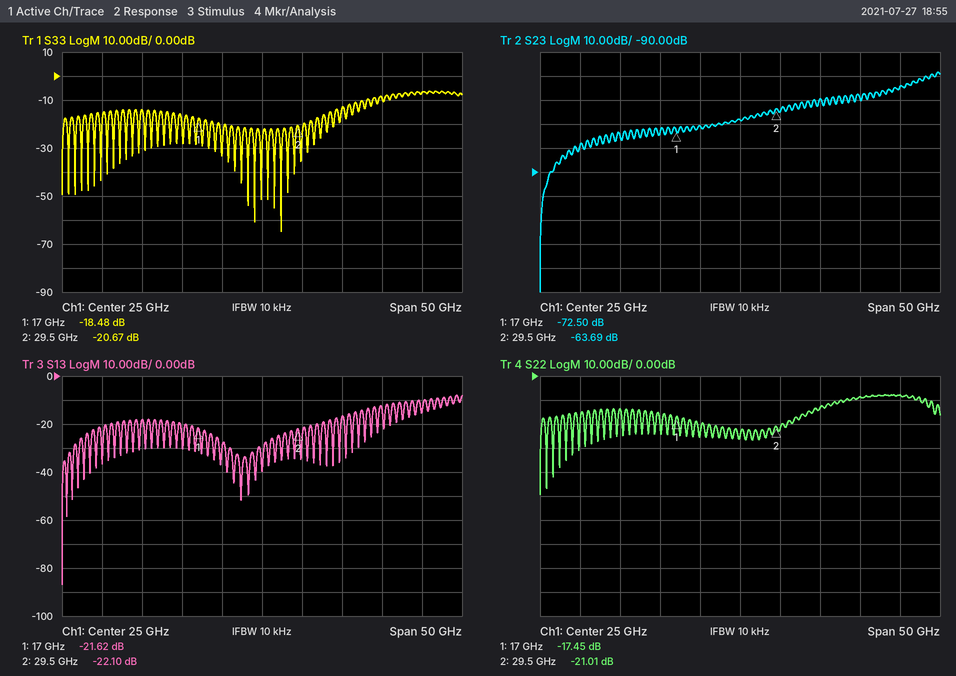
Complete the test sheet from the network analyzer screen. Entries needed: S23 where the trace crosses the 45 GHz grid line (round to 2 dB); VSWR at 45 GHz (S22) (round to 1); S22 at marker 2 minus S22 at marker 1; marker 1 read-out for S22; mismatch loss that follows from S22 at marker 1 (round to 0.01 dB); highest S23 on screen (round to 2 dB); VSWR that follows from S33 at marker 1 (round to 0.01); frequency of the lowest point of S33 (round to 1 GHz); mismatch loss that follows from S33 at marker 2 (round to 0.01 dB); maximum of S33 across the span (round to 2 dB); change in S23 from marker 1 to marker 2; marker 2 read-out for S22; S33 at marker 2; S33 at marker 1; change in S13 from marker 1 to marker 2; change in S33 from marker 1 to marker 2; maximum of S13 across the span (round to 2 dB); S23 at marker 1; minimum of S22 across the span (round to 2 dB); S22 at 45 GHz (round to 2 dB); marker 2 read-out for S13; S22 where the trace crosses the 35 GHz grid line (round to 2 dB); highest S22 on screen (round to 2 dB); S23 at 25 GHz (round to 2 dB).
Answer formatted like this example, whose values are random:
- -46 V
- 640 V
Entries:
- -54 dB
- 2
- -3.56 dB
- -17.45 dB
- 0.08 dB
- -48 dB
- 1.27
- 27 GHz
- 0.04 dB
- -6 dB
- 8.81 dB
- -21.01 dB
- -20.67 dB
- -18.48 dB
- -0.48 dB
- -2.19 dB
- -8 dB
- -72.50 dB
- -50 dB
- -8 dB
- -22.10 dB
- -14 dB
- -8 dB
- -68 dB
